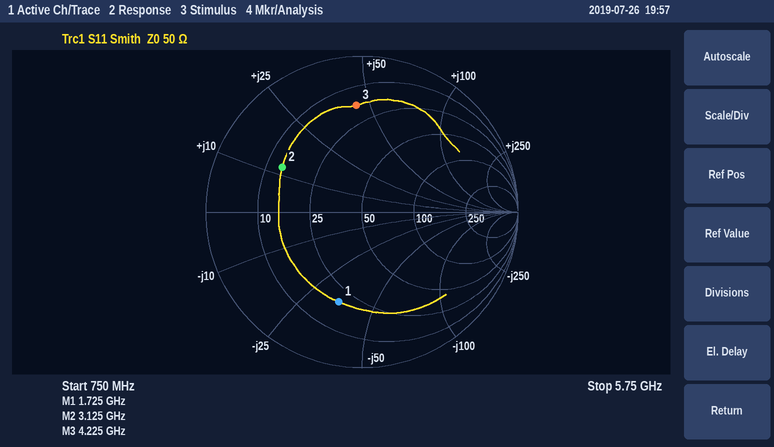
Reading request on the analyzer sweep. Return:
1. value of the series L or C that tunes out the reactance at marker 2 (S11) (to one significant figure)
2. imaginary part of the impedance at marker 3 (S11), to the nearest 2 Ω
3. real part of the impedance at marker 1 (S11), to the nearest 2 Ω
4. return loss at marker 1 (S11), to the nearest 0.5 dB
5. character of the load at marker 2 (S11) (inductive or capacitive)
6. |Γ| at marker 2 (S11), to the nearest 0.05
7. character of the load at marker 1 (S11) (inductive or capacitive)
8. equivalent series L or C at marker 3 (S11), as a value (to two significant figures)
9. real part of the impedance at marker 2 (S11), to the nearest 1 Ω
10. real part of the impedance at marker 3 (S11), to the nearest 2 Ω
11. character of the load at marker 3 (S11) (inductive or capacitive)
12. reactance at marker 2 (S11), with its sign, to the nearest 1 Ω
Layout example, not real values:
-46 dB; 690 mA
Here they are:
4 pF; +44 Ω; 20 Ω; 4.5 dB; inductive; 0.60; capacitive; 1.7 nH; 14 Ω; 18 Ω; inductive; +12 Ω
